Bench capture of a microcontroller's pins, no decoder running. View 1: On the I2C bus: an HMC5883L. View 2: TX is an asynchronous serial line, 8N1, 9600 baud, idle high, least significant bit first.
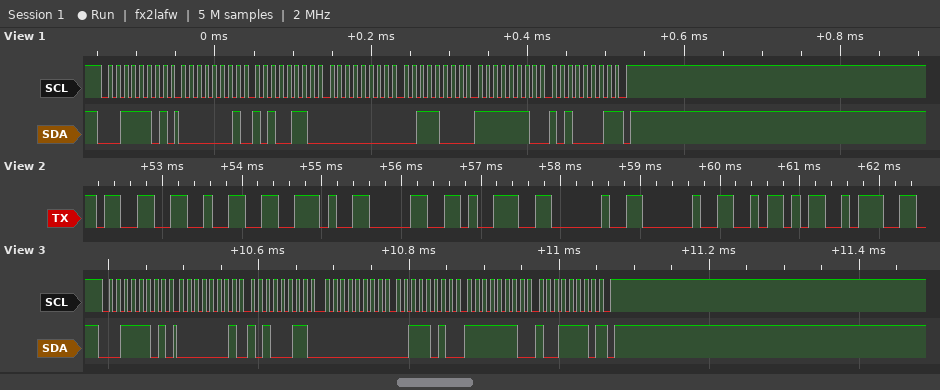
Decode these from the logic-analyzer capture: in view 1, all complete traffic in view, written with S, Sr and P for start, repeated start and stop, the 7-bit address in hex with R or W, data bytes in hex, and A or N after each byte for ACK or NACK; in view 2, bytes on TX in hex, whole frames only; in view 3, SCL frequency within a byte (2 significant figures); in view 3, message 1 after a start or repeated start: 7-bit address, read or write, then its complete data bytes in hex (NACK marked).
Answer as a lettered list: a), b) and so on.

a) S 1ER A 01 A A6 A 00 A 38 A FE A A1 N P
b) 33 32 2E 30 39 20 20 5A 3A
c) 100 kHz
d) 0x1E read: 01 A3 00 3A FE 9E NACK
